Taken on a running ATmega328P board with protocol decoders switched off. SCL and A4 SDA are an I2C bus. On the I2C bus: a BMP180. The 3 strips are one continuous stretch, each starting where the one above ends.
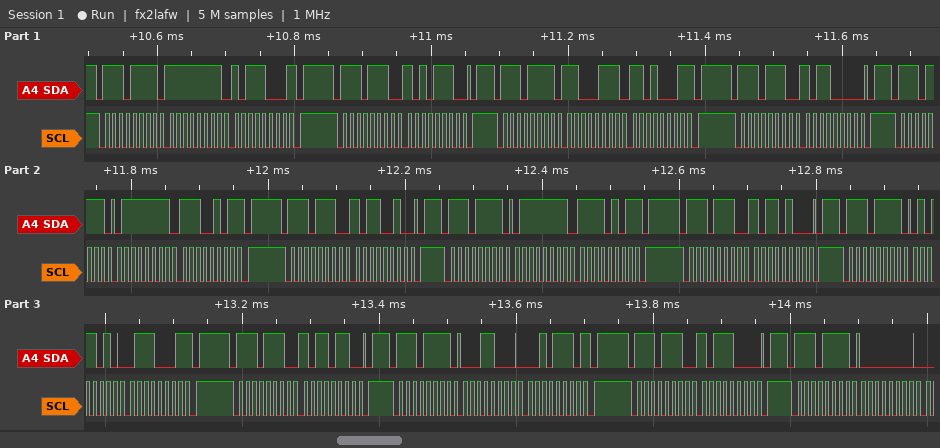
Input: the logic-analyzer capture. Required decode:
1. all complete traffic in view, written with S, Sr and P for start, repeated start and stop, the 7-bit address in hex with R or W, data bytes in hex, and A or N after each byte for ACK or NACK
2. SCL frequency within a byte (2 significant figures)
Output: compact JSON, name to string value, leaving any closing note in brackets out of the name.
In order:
{"all complete traffic in view, written with S, Sr and P for start, repeated start and stop, the 7-bit address in hex with R or W, data bytes in hex, and A or N after each byte for ACK or NACK": "S 77R A FF A B8 N P S 77W A AE A P S 77R A C7 A D1 N P S 77W A B0 A P S 77R A 7F A E5 N P S 77W A B2 A P S 77R A 7F A F5 N P S 77W A B4 A P S 77R A 5A A 71 N P S 77W A B6 A P S 77R A 18 A 2E N P S 77W A B8 A P S 77R A 00 A", "SCL frequency within a byte": "100 kHz"}
